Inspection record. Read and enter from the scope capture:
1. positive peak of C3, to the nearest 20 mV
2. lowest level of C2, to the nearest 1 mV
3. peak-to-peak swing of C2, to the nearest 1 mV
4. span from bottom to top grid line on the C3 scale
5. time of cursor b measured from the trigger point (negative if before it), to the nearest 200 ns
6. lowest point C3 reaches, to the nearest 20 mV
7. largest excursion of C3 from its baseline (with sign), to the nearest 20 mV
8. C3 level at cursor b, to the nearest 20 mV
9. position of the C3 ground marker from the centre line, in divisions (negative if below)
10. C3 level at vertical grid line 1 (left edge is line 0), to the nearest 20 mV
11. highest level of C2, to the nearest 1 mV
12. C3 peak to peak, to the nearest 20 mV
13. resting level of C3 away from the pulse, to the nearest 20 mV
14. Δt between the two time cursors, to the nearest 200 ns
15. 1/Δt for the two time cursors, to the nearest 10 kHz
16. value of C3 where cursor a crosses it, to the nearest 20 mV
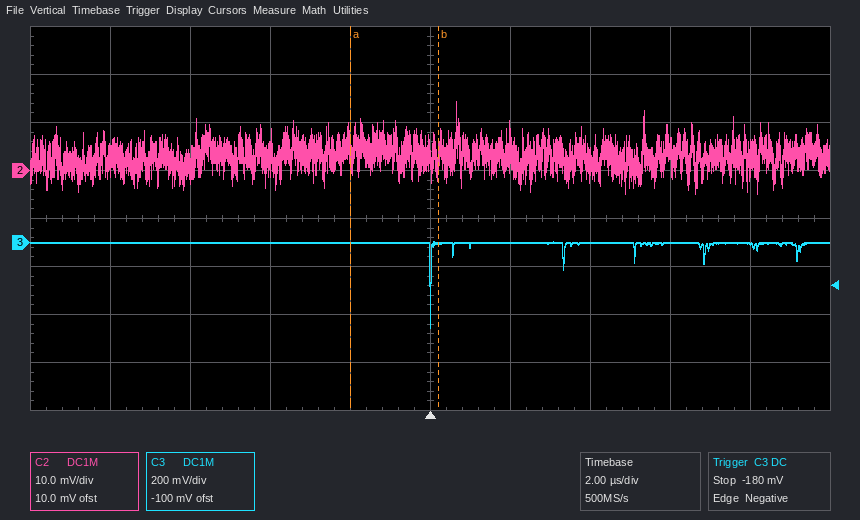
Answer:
0 mV
-5 mV
19 mV
1.6 V
+200 ns
-360 mV
-360 mV
0 mV
-0.5 div
0 mV
14 mV
360 mV
0 mV
2.2 µs
450 kHz
0 mV
